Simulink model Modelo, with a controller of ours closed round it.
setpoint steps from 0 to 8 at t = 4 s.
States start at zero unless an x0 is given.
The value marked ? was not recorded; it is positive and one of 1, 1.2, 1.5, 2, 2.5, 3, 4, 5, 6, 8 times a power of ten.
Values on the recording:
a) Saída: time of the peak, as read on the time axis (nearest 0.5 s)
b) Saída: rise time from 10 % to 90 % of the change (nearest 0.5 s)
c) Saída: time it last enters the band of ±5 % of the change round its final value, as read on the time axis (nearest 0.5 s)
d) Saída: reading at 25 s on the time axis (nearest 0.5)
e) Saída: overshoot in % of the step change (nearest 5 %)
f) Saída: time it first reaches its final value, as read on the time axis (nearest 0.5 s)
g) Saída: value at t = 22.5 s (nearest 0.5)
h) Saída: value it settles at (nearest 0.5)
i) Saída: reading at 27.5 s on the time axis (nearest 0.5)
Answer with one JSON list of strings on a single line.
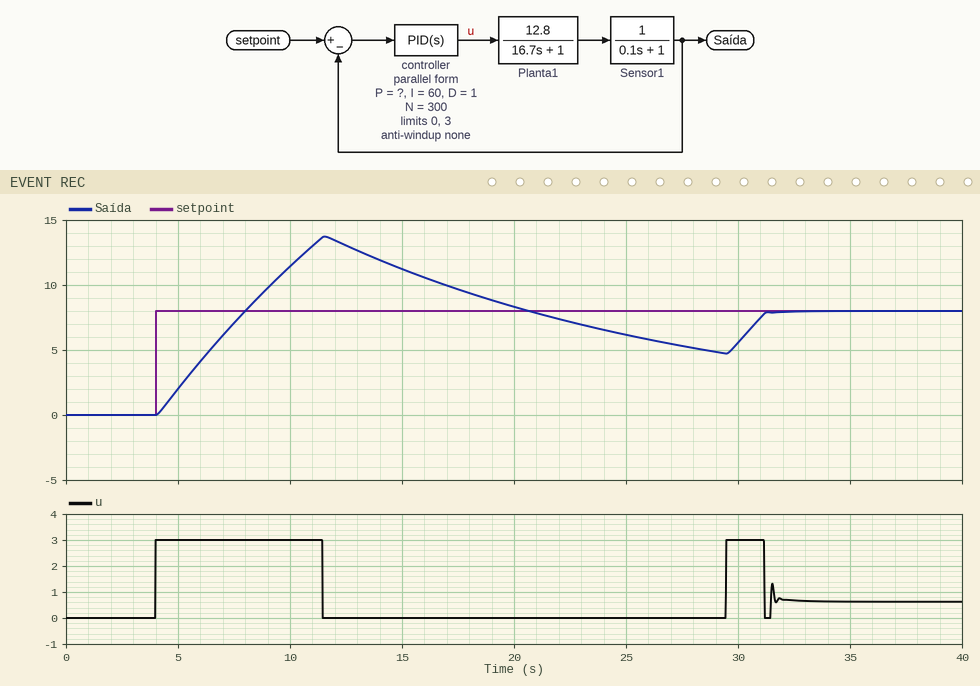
["11.5 s", "3.0 s", "31.0 s", "6.0", "70 %", "8.0 s", "7.0", "8.0", "5.5"]
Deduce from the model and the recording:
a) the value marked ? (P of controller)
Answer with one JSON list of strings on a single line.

["60"]
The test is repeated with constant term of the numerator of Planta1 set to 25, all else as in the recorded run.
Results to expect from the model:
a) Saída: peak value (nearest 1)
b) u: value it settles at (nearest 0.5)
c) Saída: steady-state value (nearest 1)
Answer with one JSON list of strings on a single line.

["13", "0.5", "8"]
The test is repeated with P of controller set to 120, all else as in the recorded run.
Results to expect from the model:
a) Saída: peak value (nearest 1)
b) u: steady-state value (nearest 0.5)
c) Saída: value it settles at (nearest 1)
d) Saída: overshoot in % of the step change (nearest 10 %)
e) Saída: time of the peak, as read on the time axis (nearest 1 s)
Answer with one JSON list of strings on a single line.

["13", "0.5", "8", "60 %", "11 s"]
